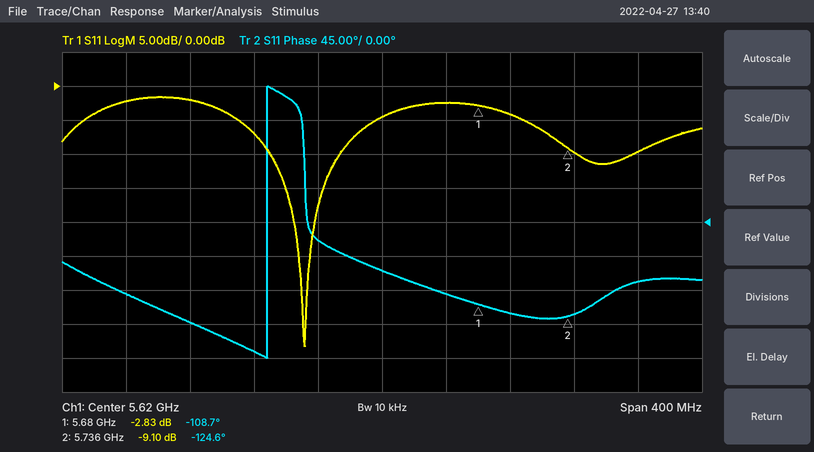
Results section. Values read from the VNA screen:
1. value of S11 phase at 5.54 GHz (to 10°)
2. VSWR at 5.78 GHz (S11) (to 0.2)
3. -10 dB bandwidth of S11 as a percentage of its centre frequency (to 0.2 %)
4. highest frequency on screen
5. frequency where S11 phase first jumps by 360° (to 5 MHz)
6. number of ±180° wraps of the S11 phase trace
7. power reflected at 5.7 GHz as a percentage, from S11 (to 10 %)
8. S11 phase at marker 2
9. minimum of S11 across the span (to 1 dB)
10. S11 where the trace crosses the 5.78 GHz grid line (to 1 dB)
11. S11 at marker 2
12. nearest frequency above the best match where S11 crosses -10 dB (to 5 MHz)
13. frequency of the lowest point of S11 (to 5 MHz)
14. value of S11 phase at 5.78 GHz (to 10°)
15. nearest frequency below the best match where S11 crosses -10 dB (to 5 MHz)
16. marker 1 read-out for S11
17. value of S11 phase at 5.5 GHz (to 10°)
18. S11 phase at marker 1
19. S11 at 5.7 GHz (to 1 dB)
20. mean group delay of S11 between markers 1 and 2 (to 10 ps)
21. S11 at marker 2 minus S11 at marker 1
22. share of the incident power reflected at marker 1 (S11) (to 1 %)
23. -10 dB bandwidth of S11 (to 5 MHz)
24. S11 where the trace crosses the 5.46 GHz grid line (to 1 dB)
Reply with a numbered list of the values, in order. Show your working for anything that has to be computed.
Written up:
1. -170°
2. |Γ| = 10^(-10/20) = 0.3162; VSWR = (1 + 0.3162)/(1 − 0.3162) ≈ 1.92, so 2.0 to the nearest 0.2
3. 45 MHz / 5.5725 GHz ≈ 0.8 %
4. 5.82 GHz
5. 5.550 GHz
6. 1
7. 10^(-4/10) ≈ 40 %
8. -124.6°
9. -38 dB
10. -10 dB
11. -9.10 dB
12. 5.595 GHz
13. 5.570 GHz
14. -80°
15. 5.550 GHz
16. -2.83 dB
17. -130°
18. -108.7°
19. -4 dB
20. −(-124.6° − (-108.7°))/(360° × 56 MHz) ≈ 789 ps, so 790 ps to the nearest 10 ps
21. -9.1 − (-2.83) = -6.27 dB
22. 10^(-2.83/10) ≈ 52 %
23. 5.595 GHz − 5.550 GHz = 45 MHz
24. -2 dB
